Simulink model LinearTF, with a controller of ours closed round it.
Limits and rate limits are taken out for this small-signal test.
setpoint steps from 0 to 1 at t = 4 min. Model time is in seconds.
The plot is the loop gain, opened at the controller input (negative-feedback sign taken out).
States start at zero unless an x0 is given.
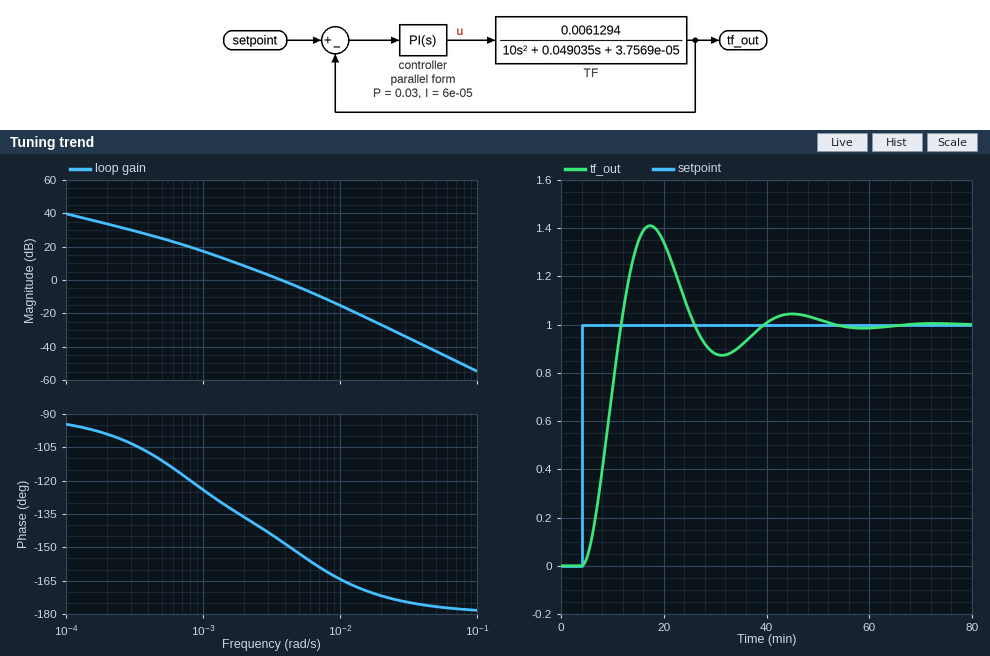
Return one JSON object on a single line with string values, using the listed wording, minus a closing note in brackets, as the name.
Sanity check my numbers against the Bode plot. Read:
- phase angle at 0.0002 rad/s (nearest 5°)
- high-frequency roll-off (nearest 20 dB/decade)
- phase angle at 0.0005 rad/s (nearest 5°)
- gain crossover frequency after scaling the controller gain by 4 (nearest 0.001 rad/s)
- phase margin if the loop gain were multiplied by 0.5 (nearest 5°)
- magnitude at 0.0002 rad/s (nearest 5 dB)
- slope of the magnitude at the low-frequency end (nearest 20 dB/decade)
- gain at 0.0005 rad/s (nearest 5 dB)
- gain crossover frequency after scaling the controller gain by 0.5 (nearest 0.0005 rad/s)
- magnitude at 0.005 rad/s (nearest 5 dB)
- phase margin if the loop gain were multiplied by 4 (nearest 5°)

{"phase angle at 0.0002 rad/s": "-100°", "high-frequency roll-off": "-40 dB/decade", "phase angle at 0.0005 rad/s": "-110°", "gain crossover frequency after scaling the controller gain by 4": "0.008 rad/s", "phase margin if the loop gain were multiplied by 0.5": "40°", "magnitude at 0.0002 rad/s": "35 dB", "slope of the magnitude at the low-frequency end": "-20 dB/decade", "gain at 0.0005 rad/s": "25 dB", "gain crossover frequency after scaling the controller gain by 0.5": "0.0025 rad/s", "magnitude at 0.005 rad/s": "-5 dB", "phase margin if the loop gain were multiplied by 4": "20°"}
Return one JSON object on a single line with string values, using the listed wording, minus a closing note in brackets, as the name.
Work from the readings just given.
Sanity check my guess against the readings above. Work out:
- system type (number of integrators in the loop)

{"system type": "1"}
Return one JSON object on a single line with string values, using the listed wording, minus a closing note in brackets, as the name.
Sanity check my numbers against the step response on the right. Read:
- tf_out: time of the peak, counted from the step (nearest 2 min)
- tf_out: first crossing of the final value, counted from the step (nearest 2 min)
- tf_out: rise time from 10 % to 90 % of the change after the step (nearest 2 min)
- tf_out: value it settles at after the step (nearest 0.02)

{"tf_out: time of the peak, counted from the step": "14 min", "tf_out: first crossing of the final value, counted from the step": "8 min", "tf_out: rise time from 10 % to 90 % of the change after the step": "6 min", "tf_out: value it settles at after the step": "1.00"}
